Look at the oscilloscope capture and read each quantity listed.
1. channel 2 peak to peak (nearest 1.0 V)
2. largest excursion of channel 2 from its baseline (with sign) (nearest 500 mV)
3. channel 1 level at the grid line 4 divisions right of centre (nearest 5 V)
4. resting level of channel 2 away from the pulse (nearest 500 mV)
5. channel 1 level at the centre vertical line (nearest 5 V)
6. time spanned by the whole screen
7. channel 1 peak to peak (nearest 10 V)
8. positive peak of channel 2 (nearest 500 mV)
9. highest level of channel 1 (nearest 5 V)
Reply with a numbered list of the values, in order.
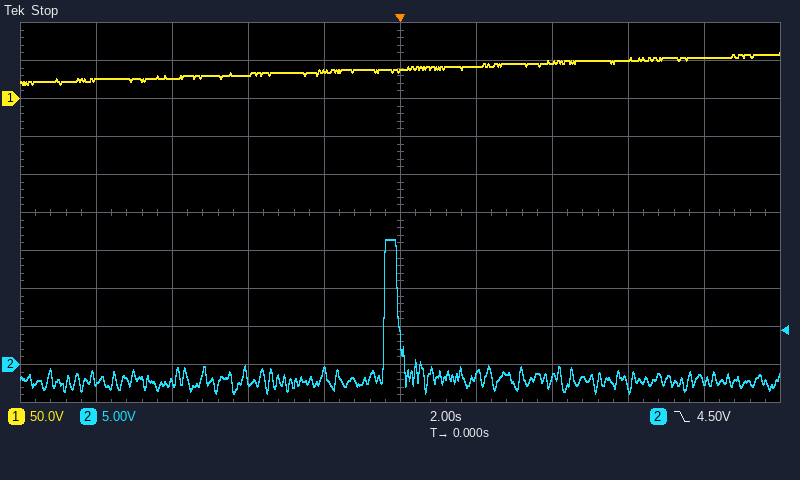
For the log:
1. 20.0 V
2. +18.5 V
3. 55 V
4. -2.0 V
5. 35 V
6. 20 s
7. 40 V
8. 16.5 V
9. 60 V
